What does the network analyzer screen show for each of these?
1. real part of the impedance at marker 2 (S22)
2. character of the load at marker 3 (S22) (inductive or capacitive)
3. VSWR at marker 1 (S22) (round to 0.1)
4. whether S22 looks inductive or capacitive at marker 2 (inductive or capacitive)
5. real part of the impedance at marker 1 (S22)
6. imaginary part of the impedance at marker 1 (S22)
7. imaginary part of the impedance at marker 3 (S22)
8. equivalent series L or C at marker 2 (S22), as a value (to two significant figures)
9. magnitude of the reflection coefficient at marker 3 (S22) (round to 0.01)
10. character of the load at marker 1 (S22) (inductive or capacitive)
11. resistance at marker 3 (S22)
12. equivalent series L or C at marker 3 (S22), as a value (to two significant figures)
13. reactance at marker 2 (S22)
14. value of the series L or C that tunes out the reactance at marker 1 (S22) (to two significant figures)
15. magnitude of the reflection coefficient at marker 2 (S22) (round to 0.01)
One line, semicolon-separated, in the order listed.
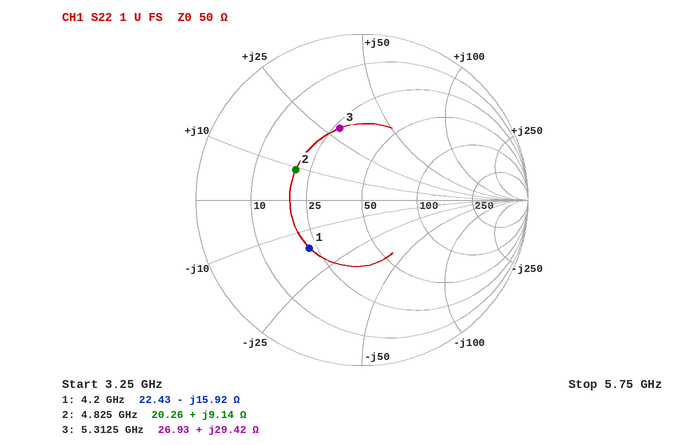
20.26 Ω; inductive; 2.5; inductive; 22.43 Ω; -15.92 Ω; +29.42 Ω; 300 pH; 0.45; capacitive; 26.93 Ω; 880 pH; +9.14 Ω; 600 pH; 0.44
